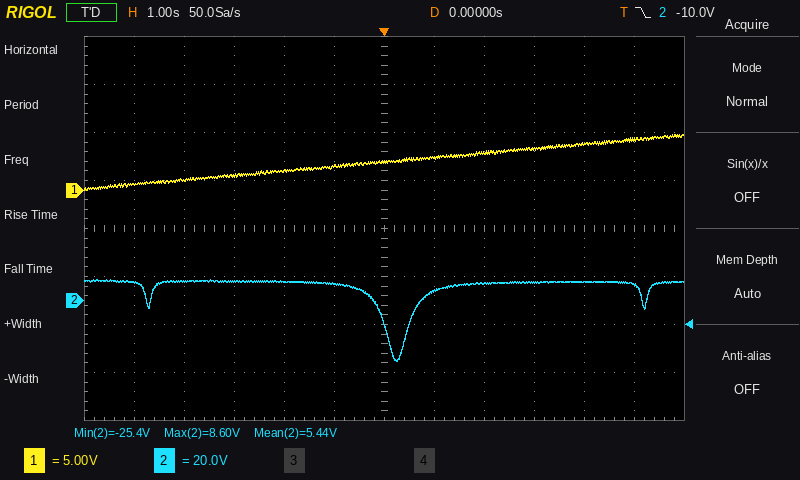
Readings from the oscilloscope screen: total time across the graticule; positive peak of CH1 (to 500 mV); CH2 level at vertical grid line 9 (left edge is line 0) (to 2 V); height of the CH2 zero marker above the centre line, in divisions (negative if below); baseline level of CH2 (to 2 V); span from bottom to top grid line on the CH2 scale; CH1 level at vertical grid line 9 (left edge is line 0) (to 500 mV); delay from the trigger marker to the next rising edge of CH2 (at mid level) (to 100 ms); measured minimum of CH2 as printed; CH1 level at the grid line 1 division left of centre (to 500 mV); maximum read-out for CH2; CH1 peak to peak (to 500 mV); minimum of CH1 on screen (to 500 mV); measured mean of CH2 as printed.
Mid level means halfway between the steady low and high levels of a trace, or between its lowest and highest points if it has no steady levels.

12 s
6.0 V
8 V
-1.5 div
8 V
160 V
4.5 V
500 ms
-25.4 V
2.5 V
8.60 V
6.0 V
0.0 V
5.44 V
